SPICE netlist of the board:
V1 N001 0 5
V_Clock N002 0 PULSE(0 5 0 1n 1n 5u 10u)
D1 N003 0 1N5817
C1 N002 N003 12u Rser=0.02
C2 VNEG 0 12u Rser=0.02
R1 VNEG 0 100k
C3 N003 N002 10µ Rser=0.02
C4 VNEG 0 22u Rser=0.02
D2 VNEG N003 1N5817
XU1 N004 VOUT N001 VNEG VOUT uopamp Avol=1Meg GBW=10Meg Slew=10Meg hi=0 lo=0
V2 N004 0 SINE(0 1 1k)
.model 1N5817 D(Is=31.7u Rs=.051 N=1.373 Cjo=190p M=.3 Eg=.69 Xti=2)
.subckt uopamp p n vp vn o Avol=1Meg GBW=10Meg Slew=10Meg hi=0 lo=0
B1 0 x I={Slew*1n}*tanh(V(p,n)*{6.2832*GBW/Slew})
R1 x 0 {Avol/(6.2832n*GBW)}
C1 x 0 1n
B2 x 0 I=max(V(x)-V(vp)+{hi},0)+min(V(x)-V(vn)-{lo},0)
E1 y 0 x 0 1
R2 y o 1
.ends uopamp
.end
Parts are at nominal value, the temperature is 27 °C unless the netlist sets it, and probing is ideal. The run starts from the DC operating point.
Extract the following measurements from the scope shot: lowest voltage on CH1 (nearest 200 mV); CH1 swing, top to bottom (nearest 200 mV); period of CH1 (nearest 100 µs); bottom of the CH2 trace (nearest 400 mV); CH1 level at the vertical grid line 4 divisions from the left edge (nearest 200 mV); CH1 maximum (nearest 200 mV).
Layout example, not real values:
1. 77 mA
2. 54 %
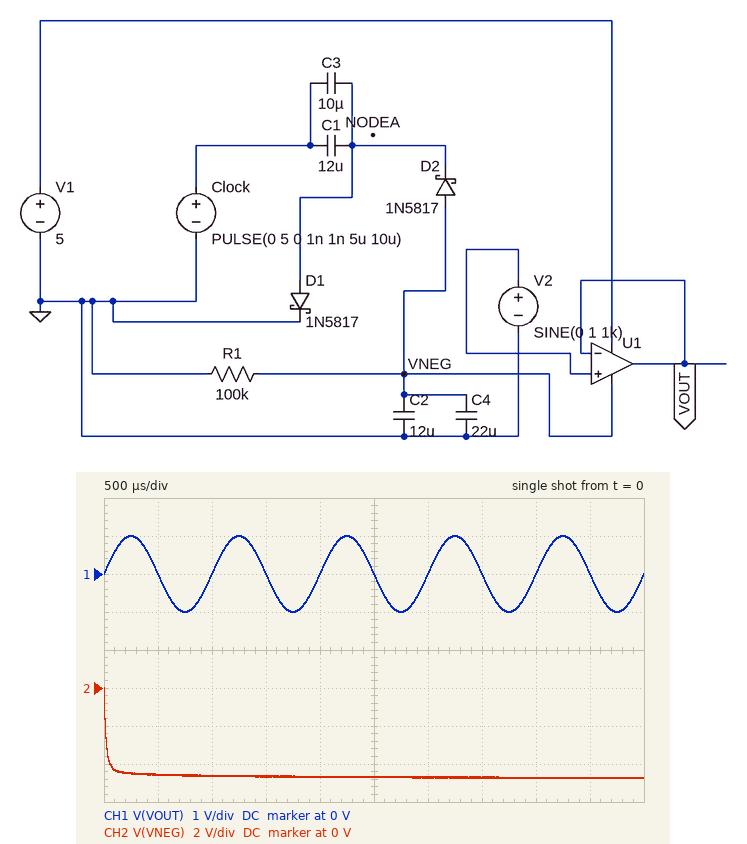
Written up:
1. -1.0 V
2. 2.0 V
3. 1.0 ms
4. -4.8 V
5. 0 V
6. 1.0 V
